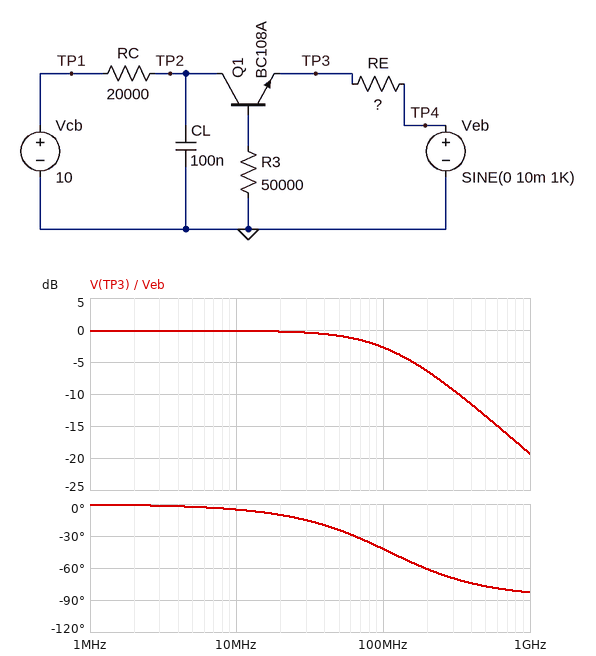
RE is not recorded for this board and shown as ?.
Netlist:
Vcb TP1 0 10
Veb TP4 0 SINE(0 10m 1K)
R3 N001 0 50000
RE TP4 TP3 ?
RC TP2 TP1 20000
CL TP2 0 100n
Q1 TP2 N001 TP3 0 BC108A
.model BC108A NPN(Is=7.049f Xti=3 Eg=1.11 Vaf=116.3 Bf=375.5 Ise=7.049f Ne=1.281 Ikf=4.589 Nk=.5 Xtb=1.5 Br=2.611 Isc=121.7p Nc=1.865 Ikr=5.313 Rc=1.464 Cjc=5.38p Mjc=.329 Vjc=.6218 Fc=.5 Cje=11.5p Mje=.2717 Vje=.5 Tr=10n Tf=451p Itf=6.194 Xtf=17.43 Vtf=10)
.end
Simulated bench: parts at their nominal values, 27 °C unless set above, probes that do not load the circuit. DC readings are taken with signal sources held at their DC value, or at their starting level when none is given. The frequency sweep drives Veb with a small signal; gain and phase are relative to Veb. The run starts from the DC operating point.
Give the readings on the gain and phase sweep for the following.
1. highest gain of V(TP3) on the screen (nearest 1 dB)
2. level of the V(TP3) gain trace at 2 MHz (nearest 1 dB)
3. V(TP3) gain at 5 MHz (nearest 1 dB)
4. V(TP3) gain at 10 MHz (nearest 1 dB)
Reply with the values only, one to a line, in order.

0 dB
0 dB
0 dB
0 dB
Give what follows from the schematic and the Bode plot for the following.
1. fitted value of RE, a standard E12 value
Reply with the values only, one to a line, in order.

820 Ω
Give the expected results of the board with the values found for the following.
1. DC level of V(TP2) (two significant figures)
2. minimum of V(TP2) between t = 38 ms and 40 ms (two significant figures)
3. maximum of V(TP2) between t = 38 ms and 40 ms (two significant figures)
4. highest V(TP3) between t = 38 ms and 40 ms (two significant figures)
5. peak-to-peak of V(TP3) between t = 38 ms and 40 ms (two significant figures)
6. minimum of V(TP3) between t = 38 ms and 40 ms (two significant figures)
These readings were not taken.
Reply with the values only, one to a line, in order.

10 V
10 V
10 V
10 mV
20 mV
-10 mV
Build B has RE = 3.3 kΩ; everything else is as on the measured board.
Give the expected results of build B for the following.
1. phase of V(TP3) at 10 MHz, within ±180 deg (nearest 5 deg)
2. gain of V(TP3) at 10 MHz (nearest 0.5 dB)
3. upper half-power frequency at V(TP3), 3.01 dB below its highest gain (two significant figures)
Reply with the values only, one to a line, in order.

-20 deg
-1.0 dB
26 MHz
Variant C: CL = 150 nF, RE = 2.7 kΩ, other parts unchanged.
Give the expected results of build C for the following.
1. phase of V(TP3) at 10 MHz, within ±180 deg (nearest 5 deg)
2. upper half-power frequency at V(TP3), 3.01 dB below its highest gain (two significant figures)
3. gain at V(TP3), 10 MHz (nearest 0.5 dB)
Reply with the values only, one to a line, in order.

-15 deg
32 MHz
-0.5 dB
